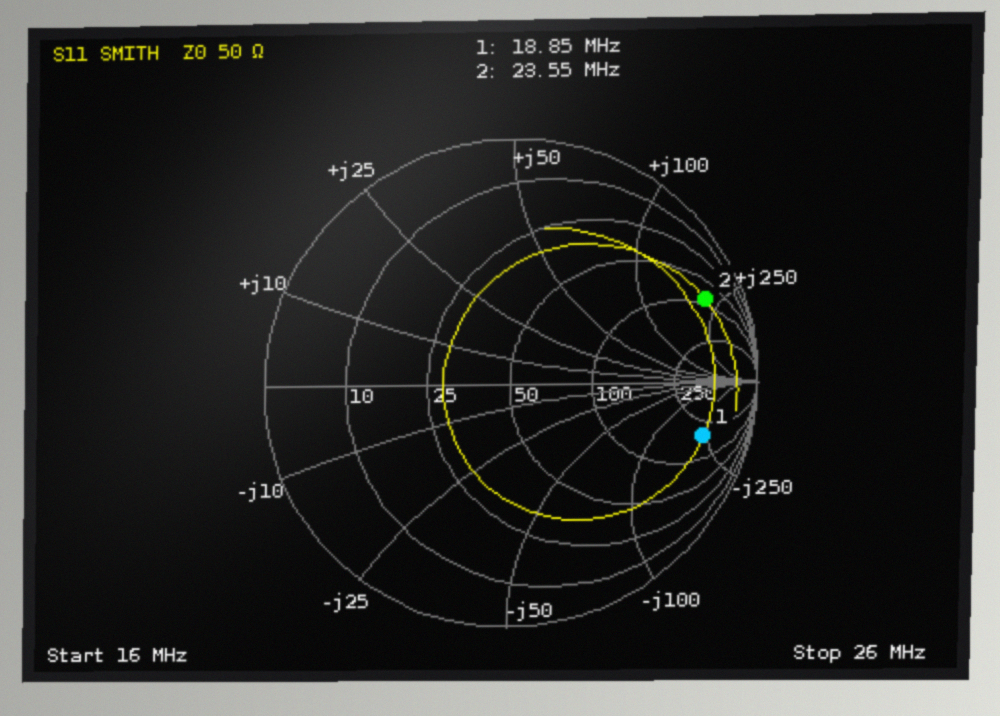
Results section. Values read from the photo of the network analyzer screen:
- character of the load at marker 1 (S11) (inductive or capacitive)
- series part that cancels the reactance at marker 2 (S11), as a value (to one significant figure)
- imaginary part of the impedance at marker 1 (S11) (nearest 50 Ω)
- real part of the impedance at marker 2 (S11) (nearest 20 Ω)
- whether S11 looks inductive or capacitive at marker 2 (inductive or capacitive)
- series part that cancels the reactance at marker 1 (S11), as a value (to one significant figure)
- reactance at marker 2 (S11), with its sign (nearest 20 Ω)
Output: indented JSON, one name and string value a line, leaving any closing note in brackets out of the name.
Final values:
{
  "character of the load at marker 1 (S11)": "capacitive",
  "series part that cancels the reactance at marker 2 (S11), as a value": "30 pF",
  "imaginary part of the impedance at marker 1 (S11)": "-250 Ω",
  "real part of the impedance at marker 2 (S11)": "80 Ω",
  "whether S11 looks inductive or capacitive at marker 2": "inductive",
  "series part that cancels the reactance at marker 1 (S11), as a value": "2 µH",
  "reactance at marker 2 (S11), with its sign": "+200 Ω"
}
